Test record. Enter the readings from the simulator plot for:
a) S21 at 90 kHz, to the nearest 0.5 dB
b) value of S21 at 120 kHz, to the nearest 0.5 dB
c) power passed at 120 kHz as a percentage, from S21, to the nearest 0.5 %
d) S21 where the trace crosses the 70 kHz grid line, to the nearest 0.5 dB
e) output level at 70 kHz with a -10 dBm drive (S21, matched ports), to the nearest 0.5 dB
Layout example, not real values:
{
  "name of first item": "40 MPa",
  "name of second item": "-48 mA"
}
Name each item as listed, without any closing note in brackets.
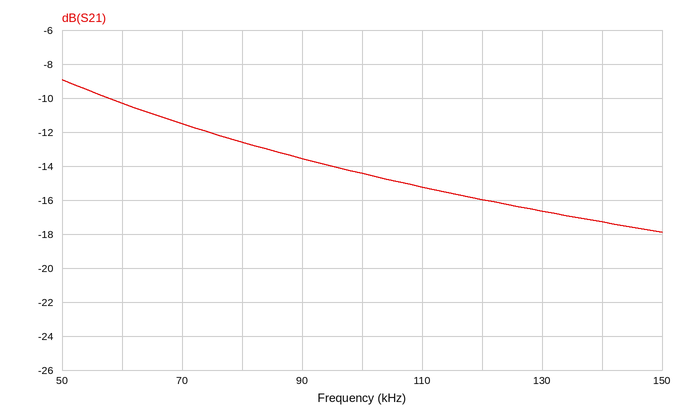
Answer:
{
  "S21 at 90 kHz, to the nearest 0.5 dB": "-13.5 dB",
  "value of S21 at 120 kHz, to the nearest 0.5 dB": "-16.0 dB",
  "power passed at 120 kHz as a percentage, from S21, to the nearest 0.5 %": "2.5 %",
  "S21 where the trace crosses the 70 kHz grid line, to the nearest 0.5 dB": "-11.5 dB",
  "output level at 70 kHz with a -10 dBm drive (S21, matched ports), to the nearest 0.5 dB": "-21.5 dBm"
}
